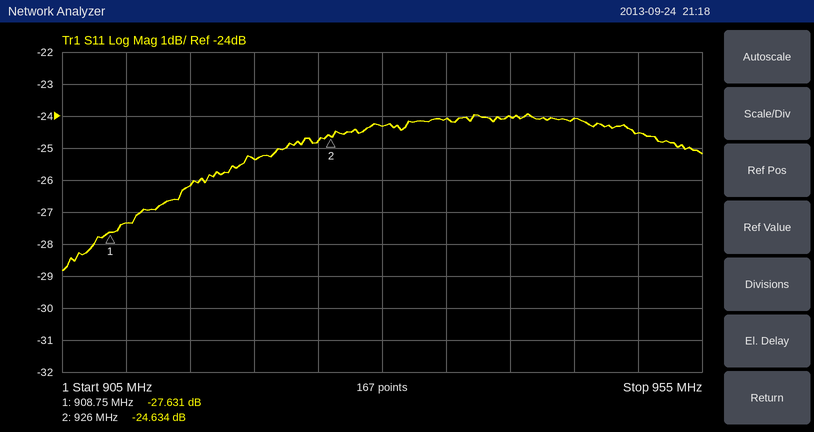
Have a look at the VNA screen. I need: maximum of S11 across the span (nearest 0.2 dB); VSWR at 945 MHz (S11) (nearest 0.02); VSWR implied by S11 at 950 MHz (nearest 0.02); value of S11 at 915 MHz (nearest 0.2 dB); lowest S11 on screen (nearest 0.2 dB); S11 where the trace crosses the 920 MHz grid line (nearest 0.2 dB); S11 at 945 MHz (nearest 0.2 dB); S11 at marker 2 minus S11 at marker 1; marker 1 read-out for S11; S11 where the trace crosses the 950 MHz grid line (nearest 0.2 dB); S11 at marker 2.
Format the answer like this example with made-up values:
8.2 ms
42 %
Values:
-24.0 dB
1.14
1.12
-26.2 dB
-28.8 dB
-25.4 dB
-24.0 dB
2.997 dB
-27.631 dB
-24.6 dB
-24.634 dB
